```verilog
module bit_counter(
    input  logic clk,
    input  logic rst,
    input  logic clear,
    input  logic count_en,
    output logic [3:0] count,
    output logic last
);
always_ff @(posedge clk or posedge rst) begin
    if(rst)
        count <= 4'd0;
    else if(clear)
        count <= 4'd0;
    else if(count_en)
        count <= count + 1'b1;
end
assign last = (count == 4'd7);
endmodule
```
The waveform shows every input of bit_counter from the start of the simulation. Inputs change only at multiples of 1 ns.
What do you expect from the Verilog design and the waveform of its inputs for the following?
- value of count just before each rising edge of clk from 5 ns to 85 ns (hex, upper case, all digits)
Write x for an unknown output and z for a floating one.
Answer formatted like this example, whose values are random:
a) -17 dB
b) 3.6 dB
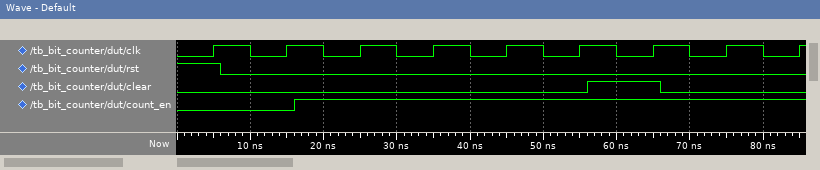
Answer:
a) 0, 0, 0, 1, 2, 3, 4, 0, 1
